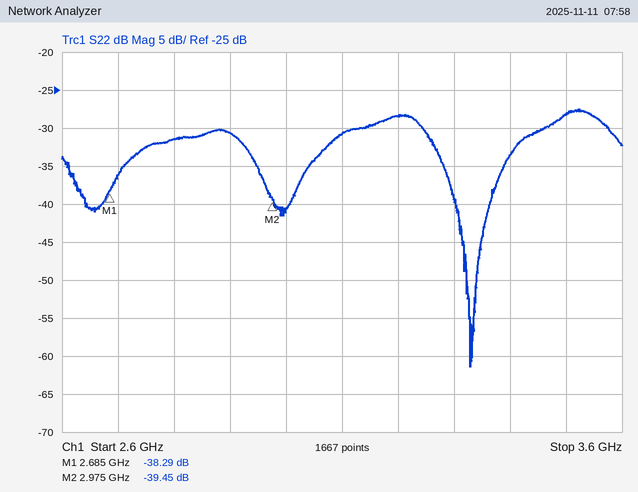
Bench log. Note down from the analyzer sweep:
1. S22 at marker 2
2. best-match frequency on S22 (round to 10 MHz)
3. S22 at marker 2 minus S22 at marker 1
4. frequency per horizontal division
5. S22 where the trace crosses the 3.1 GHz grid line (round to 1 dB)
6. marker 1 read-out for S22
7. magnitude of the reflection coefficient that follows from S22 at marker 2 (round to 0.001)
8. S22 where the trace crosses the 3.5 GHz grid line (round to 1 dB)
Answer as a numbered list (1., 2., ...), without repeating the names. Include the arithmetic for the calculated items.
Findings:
1. -39.45 dB
2. 3.33 GHz
3. -39.45 − (-38.29) = -1.16 dB
4. 100 MHz
5. -31 dB
6. -38.29 dB
7. 10^(-39.45/20) ≈ 0.011
8. -28 dB
